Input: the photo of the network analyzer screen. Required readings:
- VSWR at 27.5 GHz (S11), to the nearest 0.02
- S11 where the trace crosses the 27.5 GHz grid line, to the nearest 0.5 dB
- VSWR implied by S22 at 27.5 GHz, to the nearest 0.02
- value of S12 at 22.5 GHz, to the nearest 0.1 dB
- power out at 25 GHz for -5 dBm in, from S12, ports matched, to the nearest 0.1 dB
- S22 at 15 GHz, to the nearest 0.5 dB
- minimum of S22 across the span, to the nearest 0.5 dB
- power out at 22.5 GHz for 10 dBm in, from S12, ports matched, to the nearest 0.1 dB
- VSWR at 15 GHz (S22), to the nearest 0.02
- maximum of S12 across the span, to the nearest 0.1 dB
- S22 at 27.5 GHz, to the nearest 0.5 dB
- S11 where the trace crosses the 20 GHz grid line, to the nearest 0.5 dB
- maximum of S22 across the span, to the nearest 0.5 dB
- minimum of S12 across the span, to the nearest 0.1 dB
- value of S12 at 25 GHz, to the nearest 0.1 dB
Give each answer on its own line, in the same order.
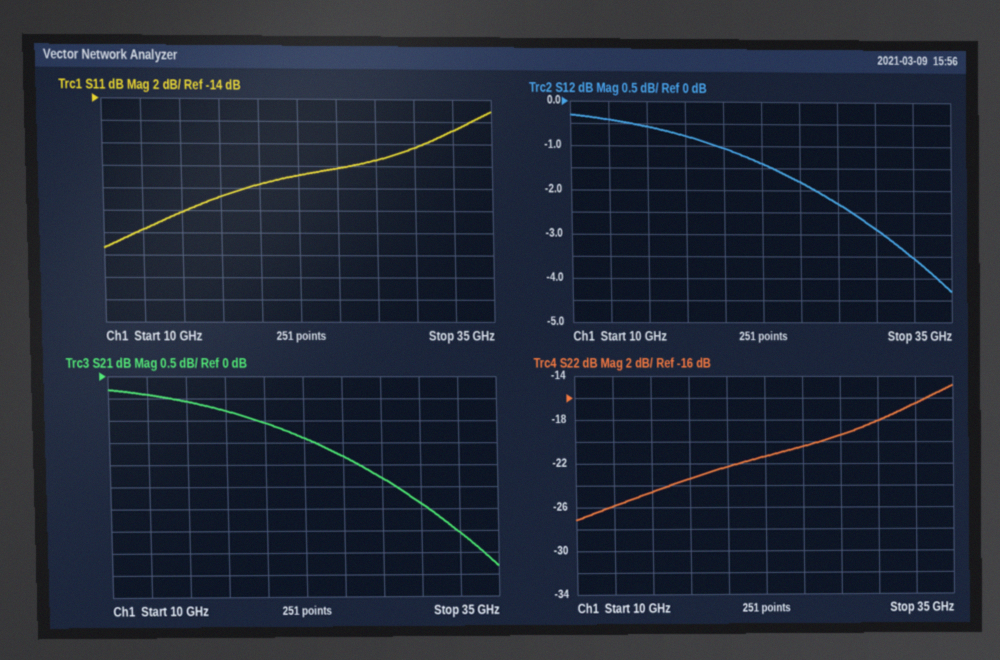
1.24
-19.5 dB
1.24
-1.4 dB
-6.8 dBm
-24.5 dB
-27.0 dB
8.6 dBm
1.12
-0.3 dB
-19.5 dB
-21.5 dB
-15.0 dB
-4.3 dB
-1.8 dB
